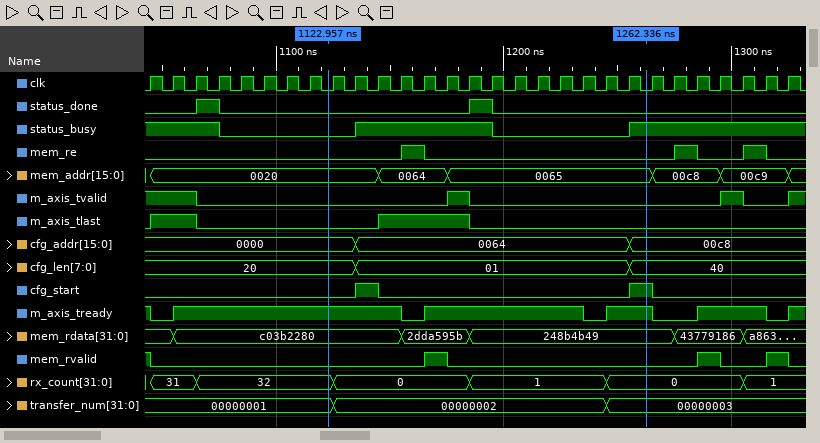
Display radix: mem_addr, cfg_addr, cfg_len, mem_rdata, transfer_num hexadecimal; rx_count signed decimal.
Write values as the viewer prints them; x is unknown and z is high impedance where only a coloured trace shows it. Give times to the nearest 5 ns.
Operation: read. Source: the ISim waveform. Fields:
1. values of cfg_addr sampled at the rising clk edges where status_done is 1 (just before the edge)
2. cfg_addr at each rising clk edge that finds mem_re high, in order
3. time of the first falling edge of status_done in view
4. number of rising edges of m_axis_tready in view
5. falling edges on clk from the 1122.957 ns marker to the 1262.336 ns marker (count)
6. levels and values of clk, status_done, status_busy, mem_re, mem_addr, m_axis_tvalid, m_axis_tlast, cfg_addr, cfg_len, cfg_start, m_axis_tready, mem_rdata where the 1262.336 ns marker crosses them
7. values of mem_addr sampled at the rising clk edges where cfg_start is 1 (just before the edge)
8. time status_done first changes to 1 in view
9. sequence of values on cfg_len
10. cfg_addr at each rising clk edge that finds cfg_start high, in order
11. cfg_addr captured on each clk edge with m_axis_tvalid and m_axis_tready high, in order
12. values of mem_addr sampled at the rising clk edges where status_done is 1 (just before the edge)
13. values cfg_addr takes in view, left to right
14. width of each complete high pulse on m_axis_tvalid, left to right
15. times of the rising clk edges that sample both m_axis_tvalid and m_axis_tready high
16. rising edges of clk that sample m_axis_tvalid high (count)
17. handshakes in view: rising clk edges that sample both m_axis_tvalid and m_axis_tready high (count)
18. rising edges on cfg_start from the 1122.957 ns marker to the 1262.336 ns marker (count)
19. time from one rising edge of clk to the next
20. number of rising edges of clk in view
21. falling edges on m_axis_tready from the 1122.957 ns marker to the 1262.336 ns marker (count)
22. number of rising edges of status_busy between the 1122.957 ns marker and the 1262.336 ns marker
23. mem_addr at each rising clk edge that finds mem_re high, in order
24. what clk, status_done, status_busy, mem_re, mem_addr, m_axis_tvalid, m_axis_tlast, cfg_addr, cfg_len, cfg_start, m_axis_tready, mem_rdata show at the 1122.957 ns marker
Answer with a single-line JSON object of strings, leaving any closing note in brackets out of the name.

{"values of cfg_addr sampled at the rising clk edges where status_done is 1": "0000, 0064", "cfg_addr at each rising clk edge that finds mem_re high, in order": "0064, 00c8, 00c8", "time of the first falling edge of status_done in view": "1075 ns", "number of rising edges of m_axis_tready in view": "5", "falling edges on clk from the 1122.957 ns marker to the 1262.336 ns marker": "14", "levels and values of clk, status_done, status_busy, mem_re, mem_addr, m_axis_tvalid, m_axis_tlast, cfg_addr, cfg_len, cfg_start, m_axis_tready, mem_rdata where the 1262.336 ns marker crosses them": "clk=0, status_done=0, status_busy=1, mem_re=0, mem_addr=0065, m_axis_tvalid=0, m_axis_tlast=0, cfg_addr=00c8, cfg_len=40, cfg_start=1, m_axis_tready=1, mem_rdata=248b4b49", "values of mem_addr sampled at the rising clk edges where cfg_start is 1": "0020, 0065", "time status_done first changes to 1 in view": "1065 ns", "sequence of values on cfg_len": "20, 01, 40", "cfg_addr at each rising clk edge that finds cfg_start high, in order": "0064, 00c8", "cfg_addr captured on each clk edge with m_axis_tvalid and m_axis_tready high, in order": "0000, 0000, 0064, 00c8", "values of mem_addr sampled at the rising clk edges where status_done is 1": "0020, 0065", "values cfg_addr takes in view, left to right": "0000, 0064, 00c8", "width of each complete high pulse on m_axis_tvalid, left to right": "10 ns, 10 ns", "times of the rising clk edges that sample both m_axis_tvalid and m_axis_tready high": "1045 ns, 1065 ns, 1185 ns, 1305 ns", "rising edges of clk that sample m_axis_tvalid high": "5", "handshakes in view: rising clk edges that sample both m_axis_tvalid and m_axis_tready high": "4", "rising edges on cfg_start from the 1122.957 ns marker to the 1262.336 ns marker": "2", "time from one rising edge of clk to the next": "10 ns", "number of rising edges of clk in view": "29", "falling edges on m_axis_tready from the 1122.957 ns marker to the 1262.336 ns marker": "2", "number of rising edges of status_busy between the 1122.957 ns marker and the 1262.336 ns marker": "2", "mem_addr at each rising clk edge that finds mem_re high, in order": "0064, 00c8, 00c9", "what clk, status_done, status_busy, mem_re, mem_addr, m_axis_tvalid, m_axis_tlast, cfg_addr, cfg_len, cfg_start, m_axis_tready, mem_rdata show at the 1122.957 ns marker": "clk=0, status_done=0, status_busy=0, mem_re=0, mem_addr=0020, m_axis_tvalid=0, m_axis_tlast=0, cfg_addr=0000, cfg_len=20, cfg_start=0, m_axis_tready=1, mem_rdata=c03b2280"}
